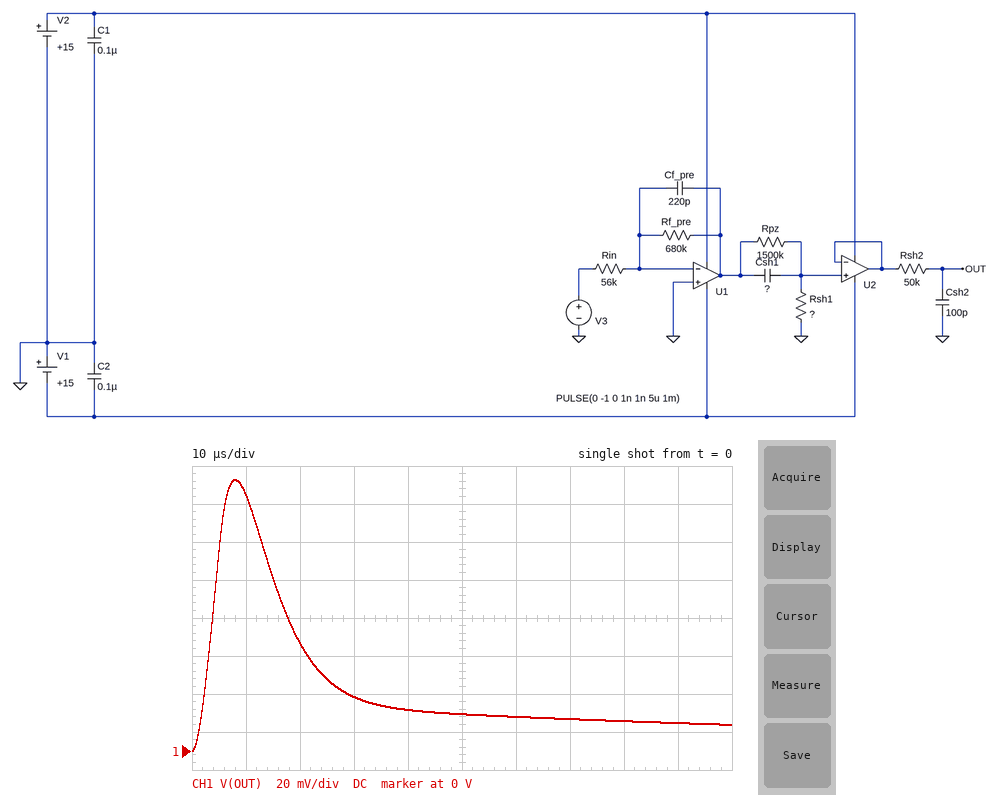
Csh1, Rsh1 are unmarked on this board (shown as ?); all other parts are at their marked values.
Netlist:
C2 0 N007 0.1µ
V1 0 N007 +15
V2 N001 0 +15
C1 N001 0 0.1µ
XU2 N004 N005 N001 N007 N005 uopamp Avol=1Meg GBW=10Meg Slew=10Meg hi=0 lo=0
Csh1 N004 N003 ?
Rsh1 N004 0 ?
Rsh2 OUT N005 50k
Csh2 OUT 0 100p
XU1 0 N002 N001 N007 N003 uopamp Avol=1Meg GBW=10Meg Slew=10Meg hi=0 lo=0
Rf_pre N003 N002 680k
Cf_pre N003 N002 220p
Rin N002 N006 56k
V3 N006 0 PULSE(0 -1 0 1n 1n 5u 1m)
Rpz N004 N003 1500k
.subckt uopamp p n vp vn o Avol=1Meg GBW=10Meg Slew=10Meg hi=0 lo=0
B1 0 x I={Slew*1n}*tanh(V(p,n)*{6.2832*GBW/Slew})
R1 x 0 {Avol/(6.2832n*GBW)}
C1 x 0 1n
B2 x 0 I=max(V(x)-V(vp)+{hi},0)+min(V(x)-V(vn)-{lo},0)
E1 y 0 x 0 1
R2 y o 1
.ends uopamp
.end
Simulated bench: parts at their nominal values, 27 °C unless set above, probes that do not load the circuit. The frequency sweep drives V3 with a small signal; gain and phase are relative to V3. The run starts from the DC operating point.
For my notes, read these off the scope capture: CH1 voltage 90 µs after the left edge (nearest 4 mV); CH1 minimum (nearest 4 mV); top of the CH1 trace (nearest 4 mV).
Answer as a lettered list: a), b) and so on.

a) 16 mV
b) 0 V
c) 144 mV
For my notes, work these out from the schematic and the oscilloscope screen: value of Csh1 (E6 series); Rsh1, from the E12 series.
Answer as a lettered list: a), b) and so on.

a) 33 pF
b) 150 kΩ
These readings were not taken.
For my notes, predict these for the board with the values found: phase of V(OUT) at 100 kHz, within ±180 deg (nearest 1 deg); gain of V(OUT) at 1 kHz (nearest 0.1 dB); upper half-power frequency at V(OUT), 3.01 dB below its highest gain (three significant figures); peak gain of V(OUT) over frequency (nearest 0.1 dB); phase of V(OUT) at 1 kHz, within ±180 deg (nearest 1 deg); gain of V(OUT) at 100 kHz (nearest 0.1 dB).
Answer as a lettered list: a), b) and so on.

a) 35 deg
b) -1.5 dB
c) 1.20 kHz
d) 0.9 dB
e) 151 deg
f) -28.7 dB
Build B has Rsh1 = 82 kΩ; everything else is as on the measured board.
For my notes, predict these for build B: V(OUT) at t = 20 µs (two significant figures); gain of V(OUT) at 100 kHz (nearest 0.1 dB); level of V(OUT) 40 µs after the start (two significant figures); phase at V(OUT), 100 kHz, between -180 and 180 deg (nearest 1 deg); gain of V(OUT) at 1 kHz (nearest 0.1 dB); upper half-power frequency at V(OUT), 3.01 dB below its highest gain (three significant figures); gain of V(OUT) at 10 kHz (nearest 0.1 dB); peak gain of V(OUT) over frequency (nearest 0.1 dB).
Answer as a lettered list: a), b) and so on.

a) 25 mV
b) -29.6 dB
c) 12 mV
d) 47 deg
e) -6.4 dB
f) 1.20 kHz
g) -13.8 dB
h) -4.0 dB
